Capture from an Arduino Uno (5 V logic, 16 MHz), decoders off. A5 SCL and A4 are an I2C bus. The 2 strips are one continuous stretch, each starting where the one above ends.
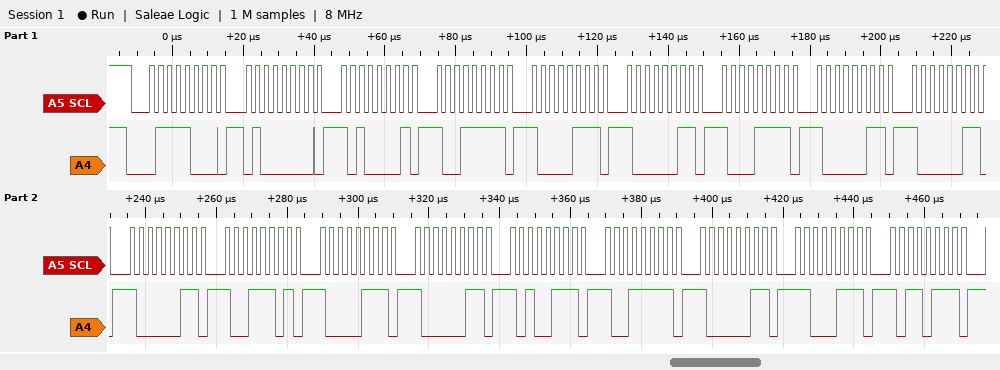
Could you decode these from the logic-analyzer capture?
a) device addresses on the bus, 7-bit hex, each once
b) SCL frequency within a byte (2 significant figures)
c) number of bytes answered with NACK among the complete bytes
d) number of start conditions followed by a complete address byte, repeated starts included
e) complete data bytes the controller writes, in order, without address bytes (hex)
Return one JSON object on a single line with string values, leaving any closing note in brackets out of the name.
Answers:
{"device addresses on the bus, 7-bit hex, each once": "0x3C", "SCL frequency within a byte": "400 kHz", "number of bytes answered with NACK among the complete bytes": "0", "number of start conditions followed by a complete address byte, repeated starts included": "1", "complete data bytes the controller writes, in order, without address bytes": "40 A1 9F 87 83 8F 83 83 83 9D 87 83 A7 9F 83 C7 B7"}
